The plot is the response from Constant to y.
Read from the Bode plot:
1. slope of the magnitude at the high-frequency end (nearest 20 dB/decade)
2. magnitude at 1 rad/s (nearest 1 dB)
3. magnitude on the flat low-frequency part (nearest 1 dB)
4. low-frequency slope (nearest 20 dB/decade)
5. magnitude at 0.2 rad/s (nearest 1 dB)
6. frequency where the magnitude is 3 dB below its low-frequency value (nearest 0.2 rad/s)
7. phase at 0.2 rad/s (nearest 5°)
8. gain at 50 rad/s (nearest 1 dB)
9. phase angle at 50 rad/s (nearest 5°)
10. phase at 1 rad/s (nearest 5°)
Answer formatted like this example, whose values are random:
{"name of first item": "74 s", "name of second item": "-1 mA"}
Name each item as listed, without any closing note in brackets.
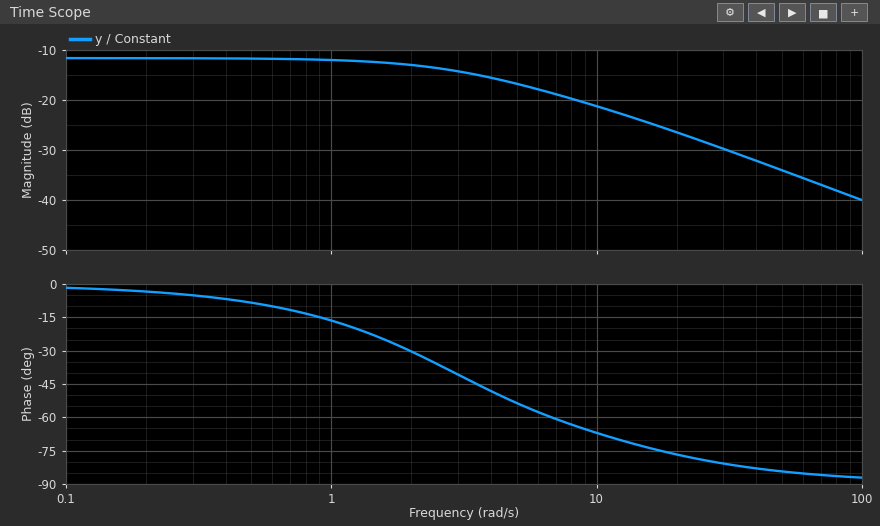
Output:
{"slope of the magnitude at the high-frequency end": "-20 dB/decade", "magnitude at 1 rad/s": "-12 dB", "magnitude on the flat low-frequency part": "-12 dB", "low-frequency slope": "0 dB/decade", "magnitude at 0.2 rad/s": "-12 dB", "frequency where the magnitude is 3 dB below its low-frequency value": "3.2 rad/s", "phase at 0.2 rad/s": "-5°", "gain at 50 rad/s": "-34 dB", "phase angle at 50 rad/s": "-85°", "phase at 1 rad/s": "-15°"}
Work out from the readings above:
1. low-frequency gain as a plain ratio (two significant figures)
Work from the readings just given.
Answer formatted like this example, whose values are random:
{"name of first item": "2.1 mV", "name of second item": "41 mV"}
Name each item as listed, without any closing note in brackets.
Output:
{"low-frequency gain as a plain ratio": "0.25"}
